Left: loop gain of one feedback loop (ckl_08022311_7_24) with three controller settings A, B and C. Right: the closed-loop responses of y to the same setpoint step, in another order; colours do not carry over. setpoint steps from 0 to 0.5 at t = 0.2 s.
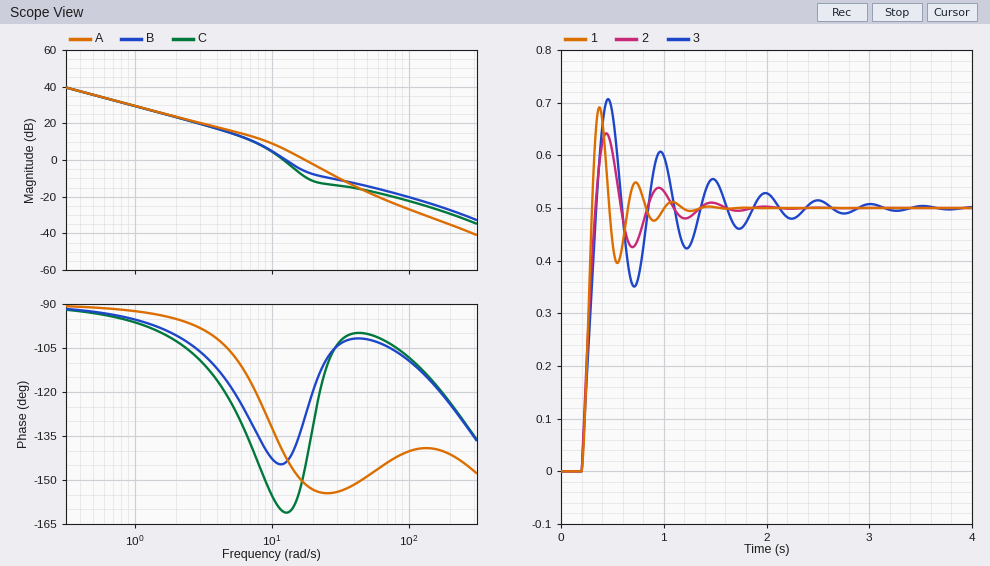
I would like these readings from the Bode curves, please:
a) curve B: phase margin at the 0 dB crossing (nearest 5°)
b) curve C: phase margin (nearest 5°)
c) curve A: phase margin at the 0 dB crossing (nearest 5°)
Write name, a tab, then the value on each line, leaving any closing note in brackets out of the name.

curve B: phase margin at the 0 dB crossing	35°
curve C: phase margin	20°
curve A: phase margin at the 0 dB crossing	30°
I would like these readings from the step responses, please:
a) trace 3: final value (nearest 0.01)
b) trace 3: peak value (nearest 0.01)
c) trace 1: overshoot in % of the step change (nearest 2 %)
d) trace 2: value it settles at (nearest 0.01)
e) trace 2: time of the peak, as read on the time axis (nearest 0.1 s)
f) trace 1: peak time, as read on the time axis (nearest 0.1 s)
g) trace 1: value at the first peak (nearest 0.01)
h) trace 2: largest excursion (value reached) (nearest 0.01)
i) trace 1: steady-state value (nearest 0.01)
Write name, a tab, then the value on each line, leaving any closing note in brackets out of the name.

trace 3: final value	0.50
trace 3: peak value	0.71
trace 1: overshoot in % of the step change	38 %
trace 2: value it settles at	0.50
trace 2: time of the peak, as read on the time axis	0.4 s
trace 1: peak time, as read on the time axis	0.4 s
trace 1: value at the first peak	0.69
trace 2: largest excursion (value reached)	0.64
trace 1: steady-state value	0.50
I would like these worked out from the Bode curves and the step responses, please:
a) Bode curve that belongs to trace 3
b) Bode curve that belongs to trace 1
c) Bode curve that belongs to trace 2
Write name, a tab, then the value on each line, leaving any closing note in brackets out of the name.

Bode curve that belongs to trace 3	C
Bode curve that belongs to trace 1	A
Bode curve that belongs to trace 2	B
